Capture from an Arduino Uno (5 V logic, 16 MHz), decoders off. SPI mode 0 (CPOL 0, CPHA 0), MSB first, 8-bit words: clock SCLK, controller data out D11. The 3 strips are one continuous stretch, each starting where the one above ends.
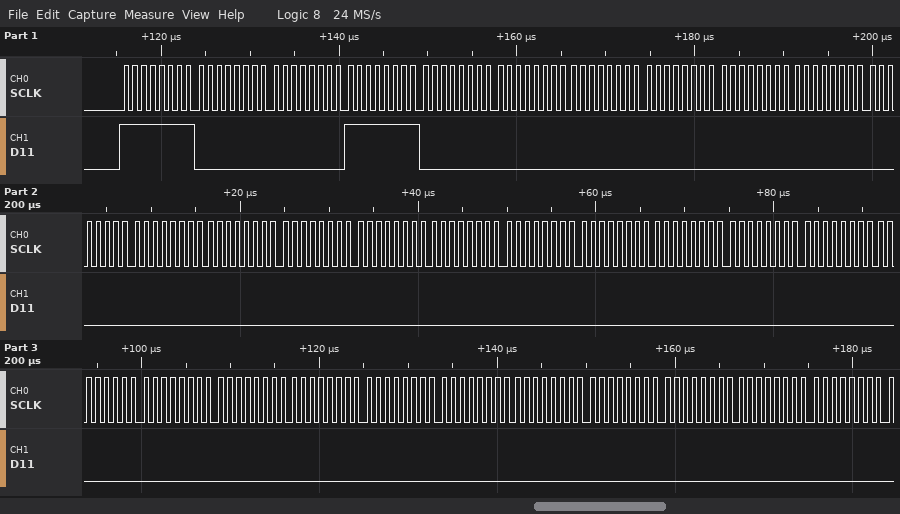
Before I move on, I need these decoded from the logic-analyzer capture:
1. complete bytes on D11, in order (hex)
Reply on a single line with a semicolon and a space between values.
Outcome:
0xFF 0x00 0x00 0xFF 0x00 0x00 0x00 0x00 0x00 0x00 0x00 0x00 0x00 0x00 0x00 0x00 0x00 0x00 0x00 0x00 0x00 0x00 0x00 0x00 0x00 0x00 0x00 0x00 0x00 0x00 0x00 0x00
